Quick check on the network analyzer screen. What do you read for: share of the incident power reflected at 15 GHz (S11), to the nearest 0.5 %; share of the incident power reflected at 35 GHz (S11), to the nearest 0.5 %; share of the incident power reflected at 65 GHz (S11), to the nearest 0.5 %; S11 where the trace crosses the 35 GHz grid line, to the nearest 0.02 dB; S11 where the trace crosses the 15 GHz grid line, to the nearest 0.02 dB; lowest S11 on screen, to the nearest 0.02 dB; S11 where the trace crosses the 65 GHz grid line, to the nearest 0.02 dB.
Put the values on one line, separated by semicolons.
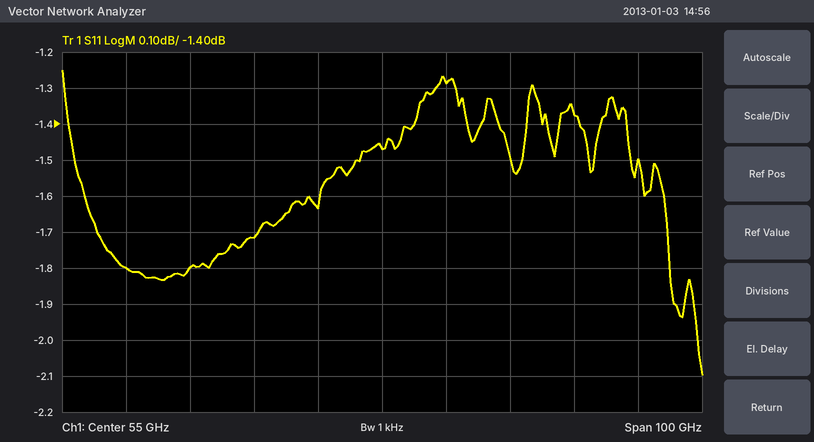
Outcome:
66.0 %; 67.5 %; 74.5 %; -1.72 dB; -1.80 dB; -2.10 dB; -1.28 dB
